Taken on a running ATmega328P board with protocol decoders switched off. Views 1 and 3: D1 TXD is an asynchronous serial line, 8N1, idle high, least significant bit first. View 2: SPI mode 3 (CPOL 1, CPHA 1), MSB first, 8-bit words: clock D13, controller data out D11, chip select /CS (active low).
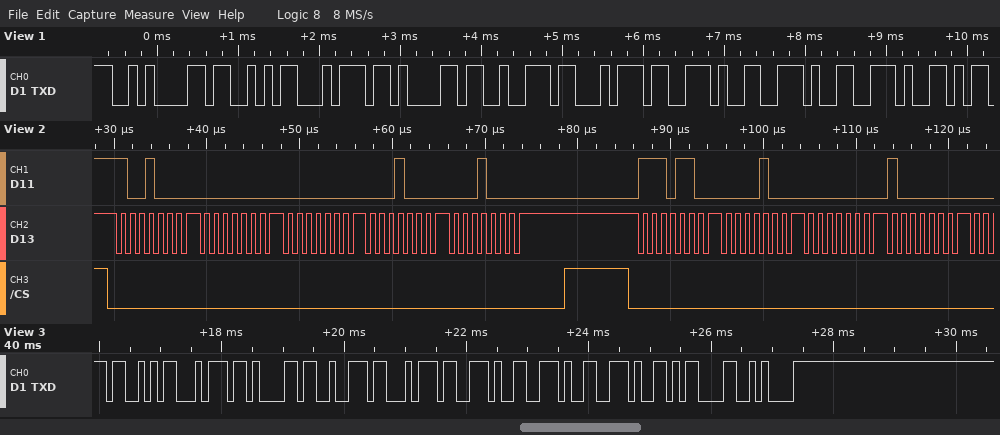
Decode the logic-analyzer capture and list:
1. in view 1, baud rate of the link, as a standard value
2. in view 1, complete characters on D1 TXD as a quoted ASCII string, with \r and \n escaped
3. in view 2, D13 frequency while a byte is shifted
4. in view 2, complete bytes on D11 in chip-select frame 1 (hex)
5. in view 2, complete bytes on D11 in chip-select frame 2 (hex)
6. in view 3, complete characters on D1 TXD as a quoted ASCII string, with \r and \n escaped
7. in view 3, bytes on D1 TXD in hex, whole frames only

9600 baud
"\nStart..."
1 MHz
90 00 00 10 10
EC 08 00 80
"Start...\r\n"
53 74 61 72 74 2E 2E 2E 0D 0A
